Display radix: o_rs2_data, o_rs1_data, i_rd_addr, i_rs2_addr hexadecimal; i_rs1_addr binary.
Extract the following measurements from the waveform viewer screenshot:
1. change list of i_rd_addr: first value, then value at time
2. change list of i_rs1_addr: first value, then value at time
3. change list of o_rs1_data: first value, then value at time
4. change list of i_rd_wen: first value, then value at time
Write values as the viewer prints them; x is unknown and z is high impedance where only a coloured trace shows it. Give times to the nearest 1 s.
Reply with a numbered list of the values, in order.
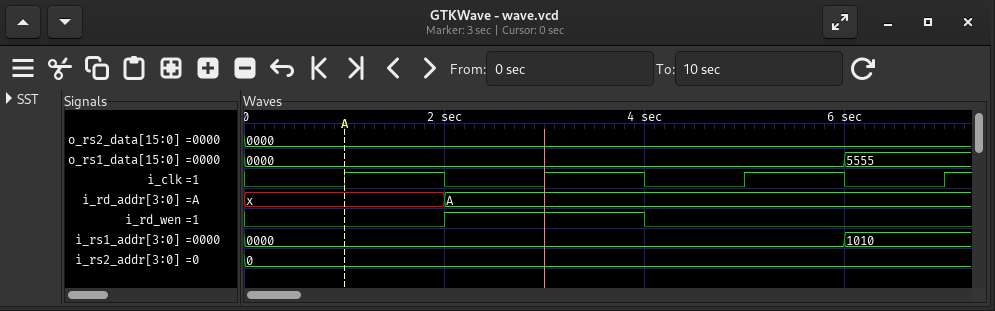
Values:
1. x, A at 2 s
2. 0000, 1010 at 6 s
3. 0000, 5555 at 6 s
4. 0, 1 at 2 s, 0 at 4 s
